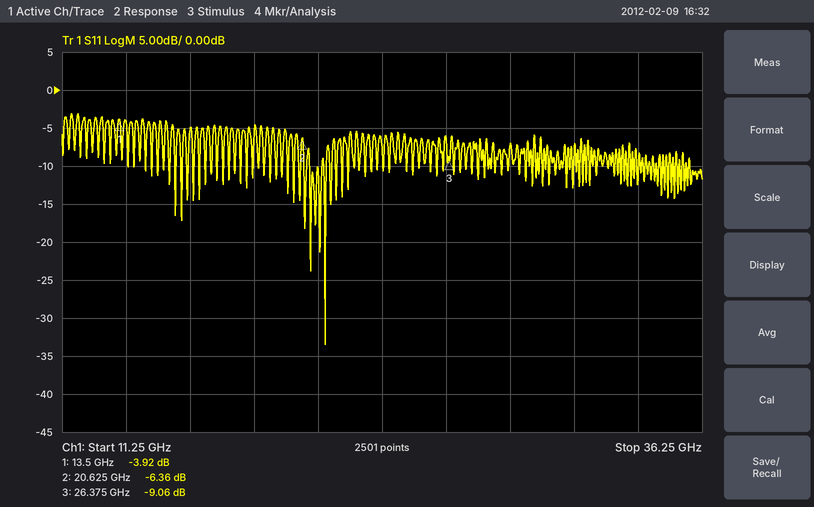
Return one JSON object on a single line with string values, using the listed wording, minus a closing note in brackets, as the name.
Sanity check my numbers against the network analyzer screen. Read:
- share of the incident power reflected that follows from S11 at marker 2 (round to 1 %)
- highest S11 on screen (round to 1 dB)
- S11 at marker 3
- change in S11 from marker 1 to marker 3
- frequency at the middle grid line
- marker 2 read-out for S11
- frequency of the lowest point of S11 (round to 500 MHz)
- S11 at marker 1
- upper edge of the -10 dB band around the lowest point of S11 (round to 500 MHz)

{"share of the incident power reflected that follows from S11 at marker 2": "23 %", "highest S11 on screen": "-3 dB", "S11 at marker 3": "-9.06 dB", "change in S11 from marker 1 to marker 3": "-5.14 dB", "frequency at the middle grid line": "23.75 GHz", "marker 2 read-out for S11": "-6.36 dB", "frequency of the lowest point of S11": "21.5 GHz", "S11 at marker 1": "-3.92 dB", "upper edge of the -10 dB band around the lowest point of S11": "21.5 GHz"}
